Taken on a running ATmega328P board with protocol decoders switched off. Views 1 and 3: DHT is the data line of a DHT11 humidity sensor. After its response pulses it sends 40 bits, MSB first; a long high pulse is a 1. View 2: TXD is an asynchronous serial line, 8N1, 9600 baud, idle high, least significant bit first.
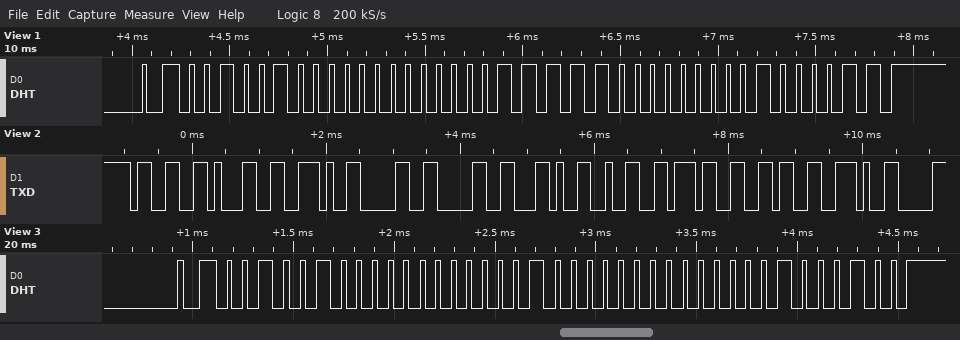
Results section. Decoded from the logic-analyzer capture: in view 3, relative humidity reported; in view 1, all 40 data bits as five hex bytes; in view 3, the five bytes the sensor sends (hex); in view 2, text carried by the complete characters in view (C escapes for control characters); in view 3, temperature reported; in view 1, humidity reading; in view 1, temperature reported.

36 %
24 00 1F 00 43
24 00 20 00 44
"31.00,276."
32.0 °C
36 %
31.0 °C
